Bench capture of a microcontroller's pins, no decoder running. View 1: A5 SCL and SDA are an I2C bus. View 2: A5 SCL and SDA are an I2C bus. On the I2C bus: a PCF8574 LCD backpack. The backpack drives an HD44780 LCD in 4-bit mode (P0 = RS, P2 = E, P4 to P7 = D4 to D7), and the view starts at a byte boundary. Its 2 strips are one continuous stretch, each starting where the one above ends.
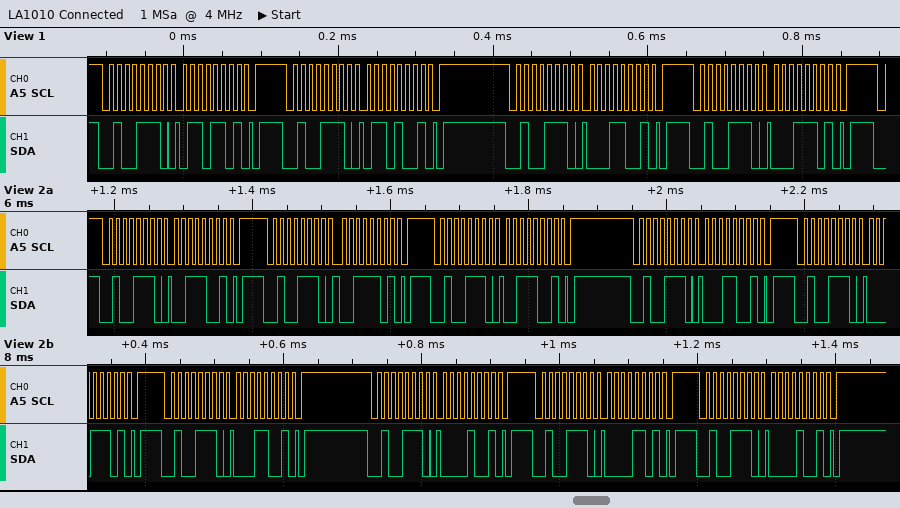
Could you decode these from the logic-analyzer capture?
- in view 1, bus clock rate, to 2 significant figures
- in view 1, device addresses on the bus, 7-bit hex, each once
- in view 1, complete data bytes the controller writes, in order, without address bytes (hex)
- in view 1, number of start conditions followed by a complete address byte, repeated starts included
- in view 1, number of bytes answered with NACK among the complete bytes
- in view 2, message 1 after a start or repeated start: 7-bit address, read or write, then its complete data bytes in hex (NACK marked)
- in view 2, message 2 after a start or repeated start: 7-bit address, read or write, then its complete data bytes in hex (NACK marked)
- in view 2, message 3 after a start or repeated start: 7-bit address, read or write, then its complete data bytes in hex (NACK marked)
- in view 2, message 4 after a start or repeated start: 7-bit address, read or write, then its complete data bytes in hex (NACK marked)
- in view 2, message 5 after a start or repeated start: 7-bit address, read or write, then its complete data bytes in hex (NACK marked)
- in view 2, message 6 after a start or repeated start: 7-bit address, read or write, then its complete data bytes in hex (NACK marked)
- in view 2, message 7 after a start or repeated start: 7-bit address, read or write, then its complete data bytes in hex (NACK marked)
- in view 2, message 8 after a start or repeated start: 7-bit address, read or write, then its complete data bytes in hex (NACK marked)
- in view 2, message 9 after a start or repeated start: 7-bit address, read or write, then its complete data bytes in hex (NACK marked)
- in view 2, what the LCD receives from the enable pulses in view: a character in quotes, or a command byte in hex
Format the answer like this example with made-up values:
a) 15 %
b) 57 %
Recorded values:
a) 100 kHz
b) 0x27
c) 6D 69 19 1D
d) 4
e) 0
f) 0x27 write: 39
g) 0x27 write: 3D
h) 0x27 write: 39
i) 0x27 write: 19
j) 0x27 write: 1D
k) 0x27 write: 19
l) 0x27 write: 09
m) 0x27 write: 0D
n) 0x27 write: 09
o) '1'
